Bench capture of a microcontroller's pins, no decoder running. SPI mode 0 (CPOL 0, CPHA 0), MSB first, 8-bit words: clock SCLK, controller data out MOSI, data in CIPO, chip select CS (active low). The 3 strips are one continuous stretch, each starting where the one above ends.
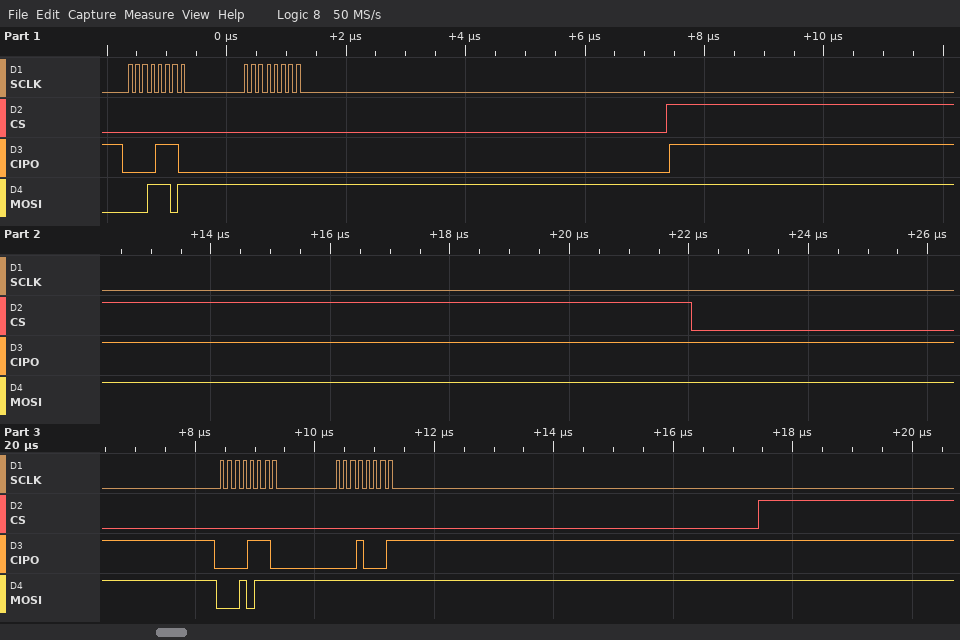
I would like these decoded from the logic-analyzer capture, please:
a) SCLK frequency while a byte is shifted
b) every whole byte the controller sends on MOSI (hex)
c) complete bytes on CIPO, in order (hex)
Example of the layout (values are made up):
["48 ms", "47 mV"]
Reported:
["8 MHz", "1D FF 17 FF", "0E 00 0E 11"]
